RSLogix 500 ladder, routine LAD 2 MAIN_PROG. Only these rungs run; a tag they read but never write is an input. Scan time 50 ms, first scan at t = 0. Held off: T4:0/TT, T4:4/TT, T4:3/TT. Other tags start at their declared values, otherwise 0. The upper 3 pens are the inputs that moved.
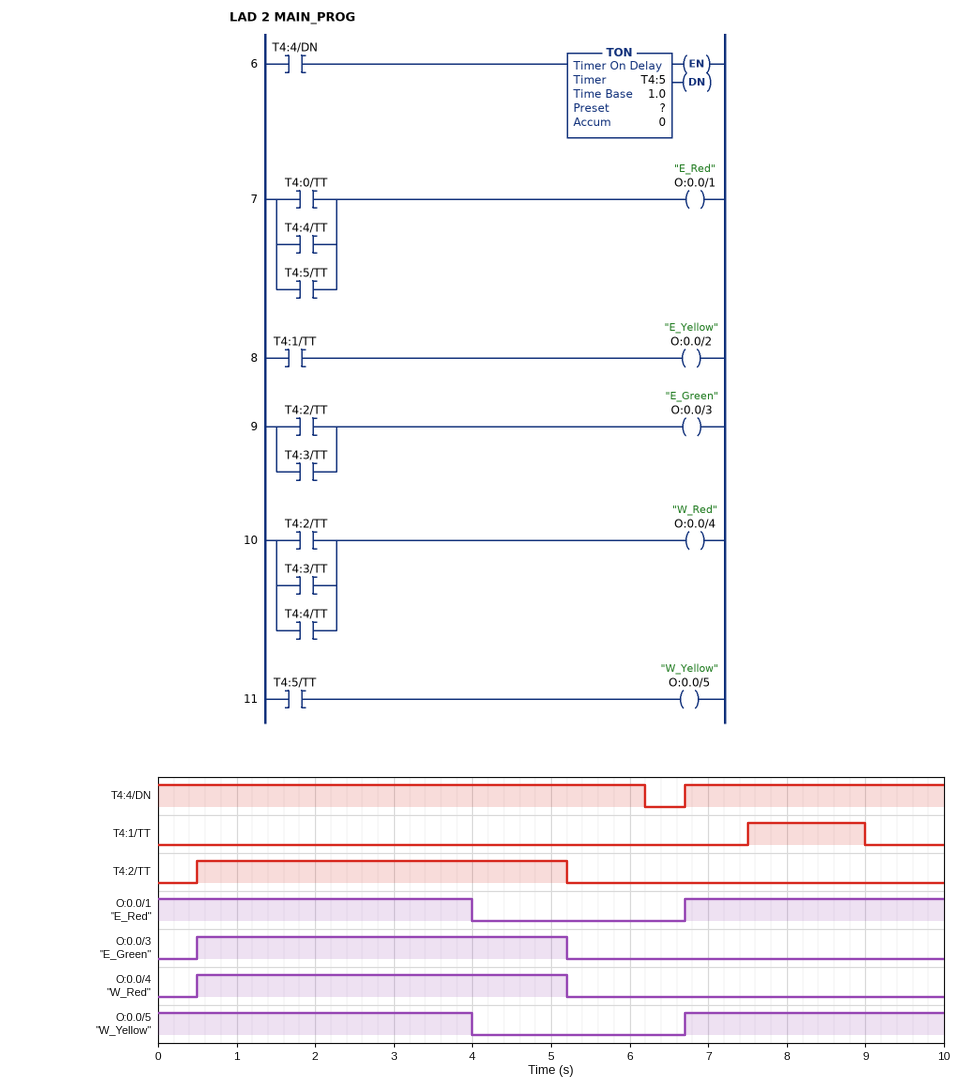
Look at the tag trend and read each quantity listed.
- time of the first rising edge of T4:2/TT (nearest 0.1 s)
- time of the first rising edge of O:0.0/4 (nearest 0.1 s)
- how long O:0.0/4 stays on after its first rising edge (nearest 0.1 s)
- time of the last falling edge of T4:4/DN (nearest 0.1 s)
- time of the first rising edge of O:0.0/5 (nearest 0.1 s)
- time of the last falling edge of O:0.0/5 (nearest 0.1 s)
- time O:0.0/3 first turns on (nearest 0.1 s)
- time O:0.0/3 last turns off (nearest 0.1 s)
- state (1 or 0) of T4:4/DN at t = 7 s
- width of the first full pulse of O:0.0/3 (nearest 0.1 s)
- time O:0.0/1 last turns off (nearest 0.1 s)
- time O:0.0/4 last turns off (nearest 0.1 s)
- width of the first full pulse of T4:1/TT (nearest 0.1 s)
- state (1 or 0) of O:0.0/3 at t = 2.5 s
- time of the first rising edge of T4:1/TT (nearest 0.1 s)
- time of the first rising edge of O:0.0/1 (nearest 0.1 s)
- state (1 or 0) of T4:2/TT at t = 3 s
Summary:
0.5 s
0.5 s
4.7 s
6.2 s
6.7 s
4.0 s
0.5 s
5.2 s
1
4.7 s
4.0 s
5.2 s
1.5 s
1
7.5 s
6.7 s
1
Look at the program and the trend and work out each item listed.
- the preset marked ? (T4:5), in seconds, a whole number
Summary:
4 s
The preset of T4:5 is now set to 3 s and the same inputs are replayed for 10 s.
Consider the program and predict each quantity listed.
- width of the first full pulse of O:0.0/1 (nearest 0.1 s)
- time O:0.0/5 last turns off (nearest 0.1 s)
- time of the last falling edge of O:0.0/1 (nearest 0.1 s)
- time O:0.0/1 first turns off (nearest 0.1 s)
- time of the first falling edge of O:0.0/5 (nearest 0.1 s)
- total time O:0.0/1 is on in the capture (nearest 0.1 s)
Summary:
3.0 s
9.7 s
9.7 s
3.0 s
3.0 s
6.0 s
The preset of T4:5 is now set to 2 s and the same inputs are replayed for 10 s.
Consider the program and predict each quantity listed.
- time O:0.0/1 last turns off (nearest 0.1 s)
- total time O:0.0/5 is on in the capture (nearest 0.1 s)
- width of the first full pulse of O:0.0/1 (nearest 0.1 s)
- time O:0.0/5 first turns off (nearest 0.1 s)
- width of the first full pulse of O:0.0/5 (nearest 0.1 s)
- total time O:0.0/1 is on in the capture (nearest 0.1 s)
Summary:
8.7 s
4.0 s
2.0 s
2.0 s
2.0 s
4.0 s
